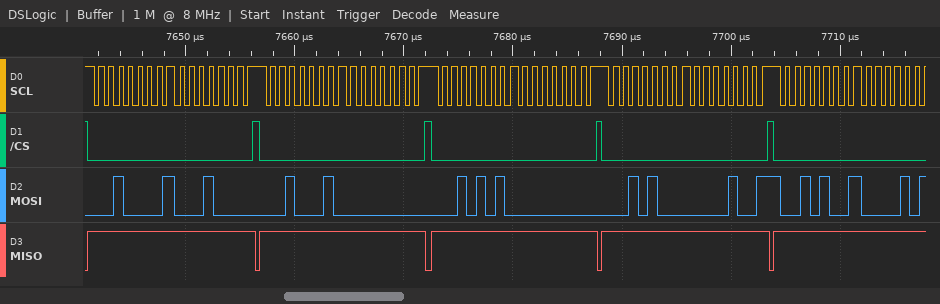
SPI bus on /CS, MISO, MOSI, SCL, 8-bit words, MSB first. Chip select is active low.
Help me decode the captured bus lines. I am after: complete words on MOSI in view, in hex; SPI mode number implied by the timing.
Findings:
21, 10, 22, 00, 2A, 00, 28, 09, 29
3
